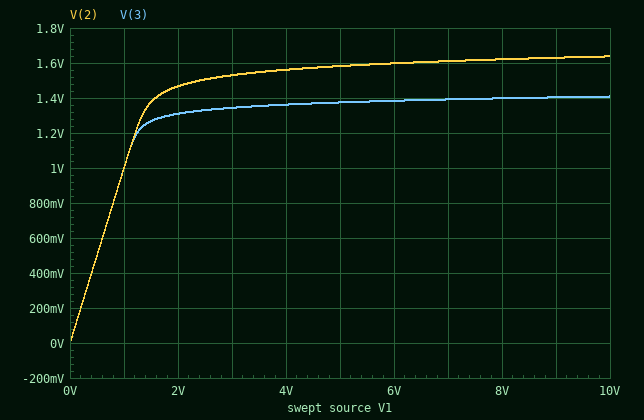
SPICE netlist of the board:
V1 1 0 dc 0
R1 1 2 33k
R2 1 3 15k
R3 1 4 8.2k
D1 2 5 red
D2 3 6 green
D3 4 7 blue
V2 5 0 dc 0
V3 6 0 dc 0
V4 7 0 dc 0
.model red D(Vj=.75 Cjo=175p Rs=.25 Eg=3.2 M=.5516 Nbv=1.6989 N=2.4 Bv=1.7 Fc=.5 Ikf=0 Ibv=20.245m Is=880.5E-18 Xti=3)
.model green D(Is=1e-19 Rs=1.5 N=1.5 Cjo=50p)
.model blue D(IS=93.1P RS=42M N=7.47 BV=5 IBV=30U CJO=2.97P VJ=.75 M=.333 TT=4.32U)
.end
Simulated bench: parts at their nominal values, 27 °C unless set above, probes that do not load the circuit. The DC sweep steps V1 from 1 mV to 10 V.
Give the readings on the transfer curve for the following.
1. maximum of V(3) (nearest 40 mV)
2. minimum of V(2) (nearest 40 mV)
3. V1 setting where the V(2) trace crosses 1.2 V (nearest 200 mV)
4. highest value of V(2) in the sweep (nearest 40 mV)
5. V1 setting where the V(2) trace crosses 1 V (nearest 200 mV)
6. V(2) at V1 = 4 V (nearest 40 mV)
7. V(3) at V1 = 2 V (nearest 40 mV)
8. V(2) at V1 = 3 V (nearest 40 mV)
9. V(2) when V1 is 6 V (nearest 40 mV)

1.40 V
0 V
1.2 V
1.64 V
1.0 V
1.56 V
1.32 V
1.52 V
1.60 V
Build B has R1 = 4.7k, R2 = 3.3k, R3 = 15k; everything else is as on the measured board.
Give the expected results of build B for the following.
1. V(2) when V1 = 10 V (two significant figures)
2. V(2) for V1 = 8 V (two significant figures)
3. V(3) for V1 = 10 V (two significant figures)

1.8 V
1.7 V
1.5 V
